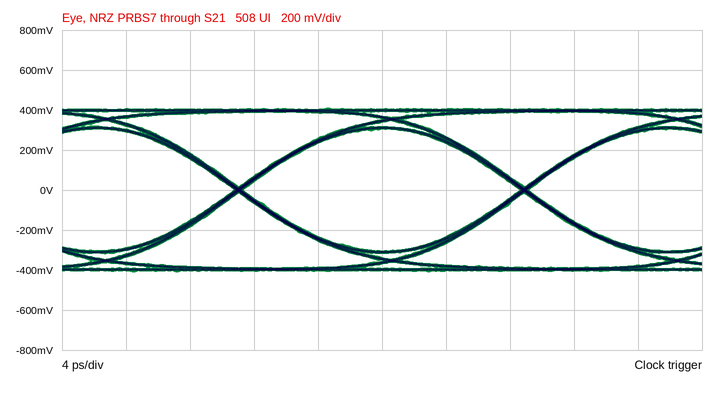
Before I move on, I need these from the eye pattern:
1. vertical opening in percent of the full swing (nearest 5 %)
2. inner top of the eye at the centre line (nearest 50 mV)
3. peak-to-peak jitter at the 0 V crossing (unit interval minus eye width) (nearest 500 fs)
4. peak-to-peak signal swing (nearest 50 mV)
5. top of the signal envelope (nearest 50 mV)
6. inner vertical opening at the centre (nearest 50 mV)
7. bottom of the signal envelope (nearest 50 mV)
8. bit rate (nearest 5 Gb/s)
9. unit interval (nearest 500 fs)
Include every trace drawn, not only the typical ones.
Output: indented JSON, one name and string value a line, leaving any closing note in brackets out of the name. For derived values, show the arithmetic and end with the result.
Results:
{
  "vertical opening in percent of the full swing": "600 mV / 800 mV ≈ 75 %",
  "inner top of the eye at the centre line": "300 mV",
  "peak-to-peak jitter at the 0 V crossing (unit interval minus eye width)": "500 fs",
  "peak-to-peak signal swing": "800 mV",
  "top of the signal envelope": "400 mV",
  "inner vertical opening at the centre": "600 mV",
  "bottom of the signal envelope": "-400 mV",
  "bit rate": "55 Gb/s",
  "unit interval": "18.0 ps"
}
